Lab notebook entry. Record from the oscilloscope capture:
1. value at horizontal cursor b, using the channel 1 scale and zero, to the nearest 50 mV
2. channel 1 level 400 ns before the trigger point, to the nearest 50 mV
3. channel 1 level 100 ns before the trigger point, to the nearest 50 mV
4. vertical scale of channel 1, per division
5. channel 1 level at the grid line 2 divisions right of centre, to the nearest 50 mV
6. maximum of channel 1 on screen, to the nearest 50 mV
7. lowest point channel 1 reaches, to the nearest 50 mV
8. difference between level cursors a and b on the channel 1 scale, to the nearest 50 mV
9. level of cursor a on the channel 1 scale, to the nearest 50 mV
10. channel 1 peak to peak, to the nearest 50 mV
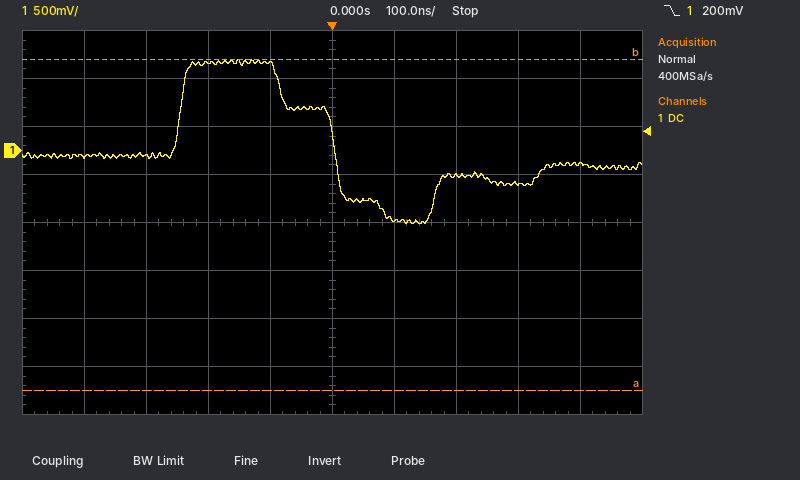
950 mV
-50 mV
900 mV
500 mV
-250 mV
950 mV
-750 mV
3.45 V
-2.50 V
1.70 V
